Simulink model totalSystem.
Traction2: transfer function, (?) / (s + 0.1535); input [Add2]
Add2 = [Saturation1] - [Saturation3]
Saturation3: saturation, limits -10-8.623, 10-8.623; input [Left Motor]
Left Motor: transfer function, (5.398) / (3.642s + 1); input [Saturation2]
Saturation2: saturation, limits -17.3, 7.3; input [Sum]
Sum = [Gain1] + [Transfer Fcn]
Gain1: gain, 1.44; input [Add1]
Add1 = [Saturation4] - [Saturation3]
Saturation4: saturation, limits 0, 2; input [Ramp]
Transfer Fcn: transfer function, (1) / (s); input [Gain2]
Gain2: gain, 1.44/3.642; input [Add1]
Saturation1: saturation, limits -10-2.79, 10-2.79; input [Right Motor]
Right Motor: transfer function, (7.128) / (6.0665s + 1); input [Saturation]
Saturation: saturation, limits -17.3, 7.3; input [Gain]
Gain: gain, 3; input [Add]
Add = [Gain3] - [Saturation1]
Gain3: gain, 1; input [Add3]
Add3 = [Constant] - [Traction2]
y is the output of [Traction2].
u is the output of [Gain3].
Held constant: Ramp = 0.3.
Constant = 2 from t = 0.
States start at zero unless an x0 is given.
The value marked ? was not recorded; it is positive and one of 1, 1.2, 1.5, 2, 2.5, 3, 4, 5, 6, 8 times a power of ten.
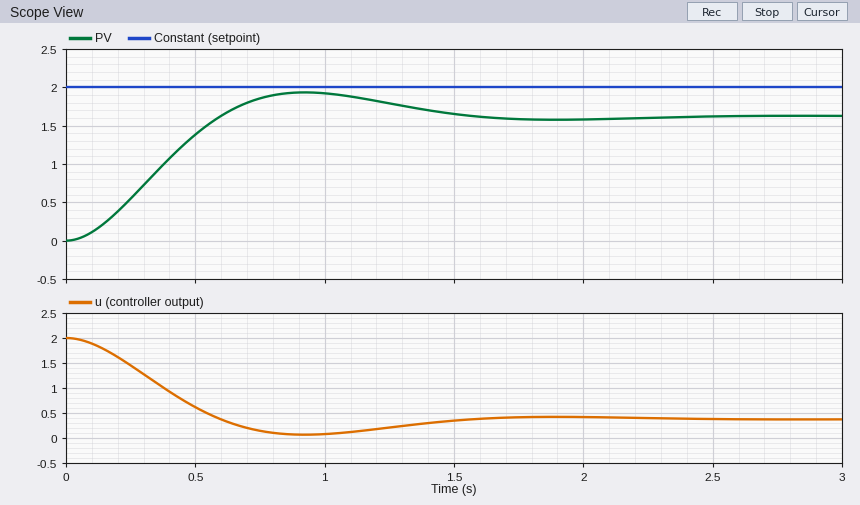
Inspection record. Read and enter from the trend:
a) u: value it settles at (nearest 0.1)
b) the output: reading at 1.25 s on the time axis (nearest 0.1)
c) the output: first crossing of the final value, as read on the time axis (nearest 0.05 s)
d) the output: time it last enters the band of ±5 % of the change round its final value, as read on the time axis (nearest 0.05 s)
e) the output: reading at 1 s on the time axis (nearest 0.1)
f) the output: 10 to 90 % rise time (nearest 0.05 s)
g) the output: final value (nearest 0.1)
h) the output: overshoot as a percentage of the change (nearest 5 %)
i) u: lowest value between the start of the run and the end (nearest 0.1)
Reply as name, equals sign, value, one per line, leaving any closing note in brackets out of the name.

u: value it settles at = 0.4
the output: reading at 1.25 s on the time axis = 1.8
the output: first crossing of the final value, as read on the time axis = 0.60 s
the output: time it last enters the band of ±5 % of the change round its final value, as read on the time axis = 1.40 s
the output: reading at 1 s on the time axis = 1.9
the output: 10 to 90 % rise time = 0.40 s
the output: final value = 1.6
the output: overshoot as a percentage of the change = 20 %
u: lowest value between the start of the run and the end = 0.1
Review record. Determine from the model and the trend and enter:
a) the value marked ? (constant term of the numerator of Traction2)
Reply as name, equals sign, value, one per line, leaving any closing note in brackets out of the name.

the value marked ? = 4
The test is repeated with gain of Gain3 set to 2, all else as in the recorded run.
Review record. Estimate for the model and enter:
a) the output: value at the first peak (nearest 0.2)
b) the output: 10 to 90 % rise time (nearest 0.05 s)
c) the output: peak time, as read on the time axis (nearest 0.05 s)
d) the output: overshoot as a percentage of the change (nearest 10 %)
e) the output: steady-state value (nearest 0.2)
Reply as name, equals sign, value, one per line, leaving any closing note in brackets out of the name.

the output: value at the first peak = 2.4
the output: 10 to 90 % rise time = 0.25 s
the output: peak time, as read on the time axis = 0.65 s
the output: overshoot as a percentage of the change = 30 %
the output: steady-state value = 1.8
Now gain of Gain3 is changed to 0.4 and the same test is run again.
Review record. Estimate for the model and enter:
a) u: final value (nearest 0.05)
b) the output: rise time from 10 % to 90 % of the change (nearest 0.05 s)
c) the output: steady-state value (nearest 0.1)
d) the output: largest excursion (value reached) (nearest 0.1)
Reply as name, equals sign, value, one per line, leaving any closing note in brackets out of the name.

u: final value = 0.35
the output: rise time from 10 % to 90 % of the change = 0.80 s
the output: steady-state value = 1.1
the output: largest excursion (value reached) = 1.2
